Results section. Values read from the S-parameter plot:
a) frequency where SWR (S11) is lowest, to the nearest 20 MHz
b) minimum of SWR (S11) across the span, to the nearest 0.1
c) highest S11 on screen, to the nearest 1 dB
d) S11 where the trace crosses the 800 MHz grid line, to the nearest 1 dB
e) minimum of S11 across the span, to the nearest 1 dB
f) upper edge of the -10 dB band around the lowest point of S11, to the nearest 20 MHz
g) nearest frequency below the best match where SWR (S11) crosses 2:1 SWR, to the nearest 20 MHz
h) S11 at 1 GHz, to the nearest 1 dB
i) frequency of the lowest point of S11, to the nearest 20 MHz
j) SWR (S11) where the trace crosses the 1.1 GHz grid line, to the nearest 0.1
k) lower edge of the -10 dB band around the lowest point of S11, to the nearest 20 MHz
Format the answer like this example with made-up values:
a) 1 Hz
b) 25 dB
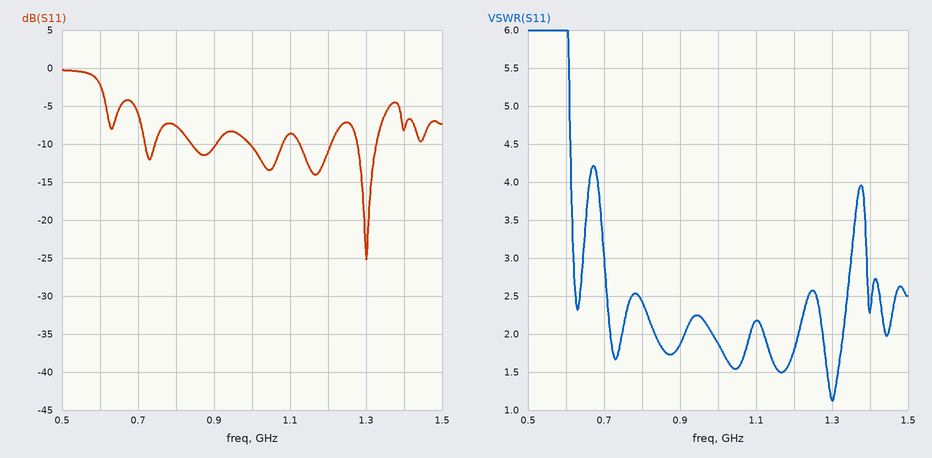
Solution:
a) 1.30 GHz
b) 1.1
c) 0 dB
d) -8 dB
e) -25 dB
f) 1.32 GHz
g) 1.28 GHz
h) -10 dB
i) 1.30 GHz
j) 2.2
k) 1.28 GHz
